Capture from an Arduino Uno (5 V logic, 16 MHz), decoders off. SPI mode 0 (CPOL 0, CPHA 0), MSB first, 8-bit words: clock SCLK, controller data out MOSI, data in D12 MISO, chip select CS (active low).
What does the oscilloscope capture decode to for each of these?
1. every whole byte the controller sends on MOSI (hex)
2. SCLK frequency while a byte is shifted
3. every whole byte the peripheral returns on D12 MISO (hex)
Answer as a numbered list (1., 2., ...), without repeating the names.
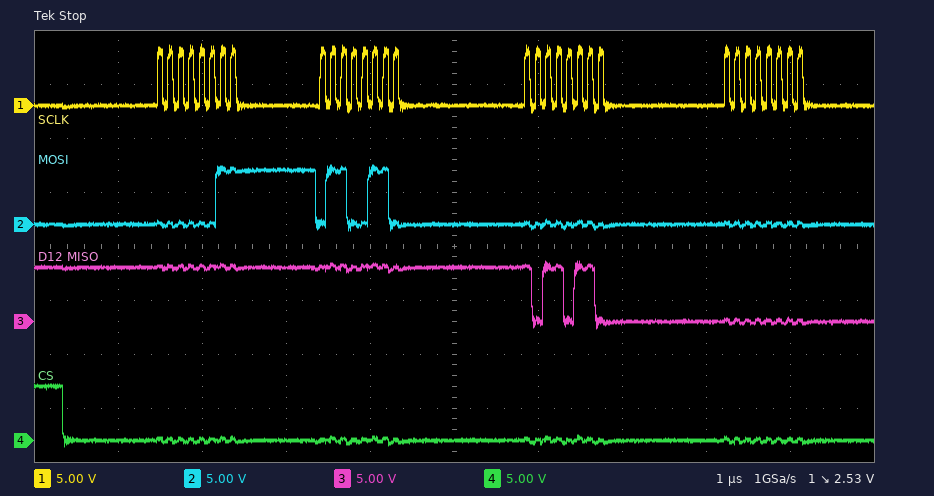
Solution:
1. 0x03 0x66 0x00 0x00
2. 8 MHz
3. 0xFF 0xFF 0xB6 0x00
